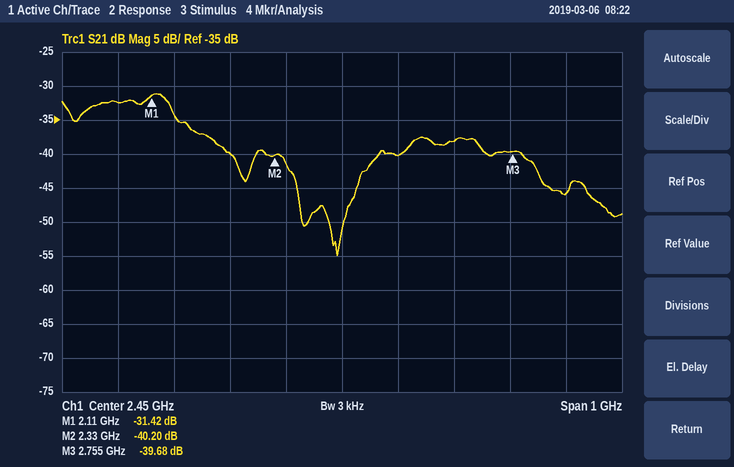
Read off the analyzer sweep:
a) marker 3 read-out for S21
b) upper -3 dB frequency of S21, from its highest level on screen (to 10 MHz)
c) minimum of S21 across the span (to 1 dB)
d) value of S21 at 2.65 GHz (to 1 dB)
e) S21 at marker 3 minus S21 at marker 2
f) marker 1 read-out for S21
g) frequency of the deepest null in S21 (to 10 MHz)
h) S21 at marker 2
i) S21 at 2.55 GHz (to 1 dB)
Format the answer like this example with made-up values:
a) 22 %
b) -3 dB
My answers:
a) -39.68 dB
b) 2.15 GHz
c) -55 dB
d) -38 dB
e) 0.52 dB
f) -31.42 dB
g) 2.44 GHz
h) -40.20 dB
i) -40 dB
